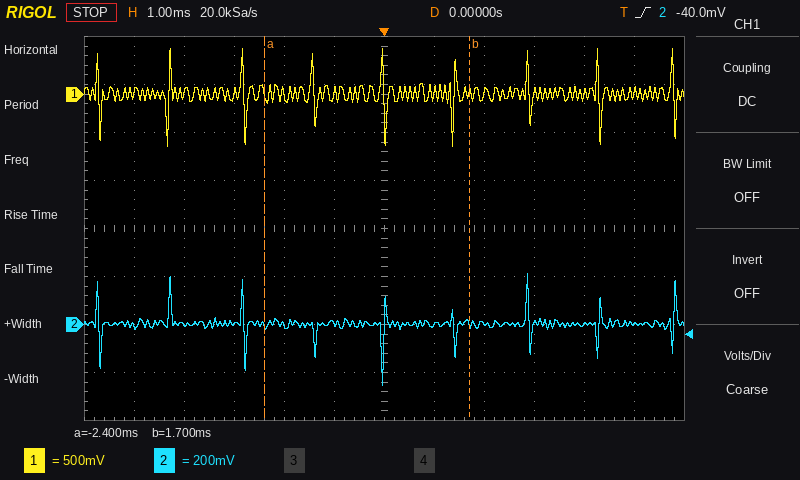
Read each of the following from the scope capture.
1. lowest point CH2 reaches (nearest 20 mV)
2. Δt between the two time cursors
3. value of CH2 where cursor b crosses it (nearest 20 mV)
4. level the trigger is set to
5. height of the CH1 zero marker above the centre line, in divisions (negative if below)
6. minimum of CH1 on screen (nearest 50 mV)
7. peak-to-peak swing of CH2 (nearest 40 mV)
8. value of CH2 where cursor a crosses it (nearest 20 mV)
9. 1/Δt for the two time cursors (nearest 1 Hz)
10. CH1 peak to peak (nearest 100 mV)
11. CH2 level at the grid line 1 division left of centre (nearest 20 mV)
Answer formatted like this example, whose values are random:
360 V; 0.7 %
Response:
-260 mV; 4.1 ms; 0 mV; -40.0 mV; +2.8 div; -550 mV; 480 mV; 0 mV; 244 Hz; 1.00 V; 0 mV
